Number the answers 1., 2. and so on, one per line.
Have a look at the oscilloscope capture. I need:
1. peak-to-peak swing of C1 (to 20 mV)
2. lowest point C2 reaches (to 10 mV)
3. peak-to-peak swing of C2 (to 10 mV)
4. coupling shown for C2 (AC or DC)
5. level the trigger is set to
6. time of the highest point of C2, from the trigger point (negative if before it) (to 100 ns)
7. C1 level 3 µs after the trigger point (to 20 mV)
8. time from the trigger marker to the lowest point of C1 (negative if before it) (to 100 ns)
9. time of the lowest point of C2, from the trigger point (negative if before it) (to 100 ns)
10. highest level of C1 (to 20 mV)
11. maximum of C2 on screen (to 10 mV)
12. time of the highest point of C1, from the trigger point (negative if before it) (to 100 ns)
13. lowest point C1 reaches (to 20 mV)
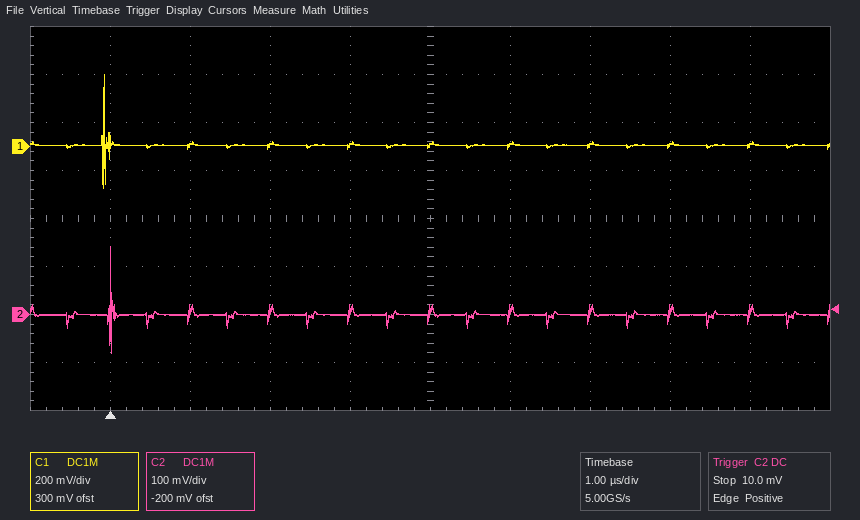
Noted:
1. 480 mV
2. -80 mV
3. 220 mV
4. DC
5. 10.0 mV
6. 0.0 µs
7. 0 mV
8. -100 ns
9. 0.0 µs
10. 300 mV
11. 140 mV
12. -100 ns
13. -180 mV
